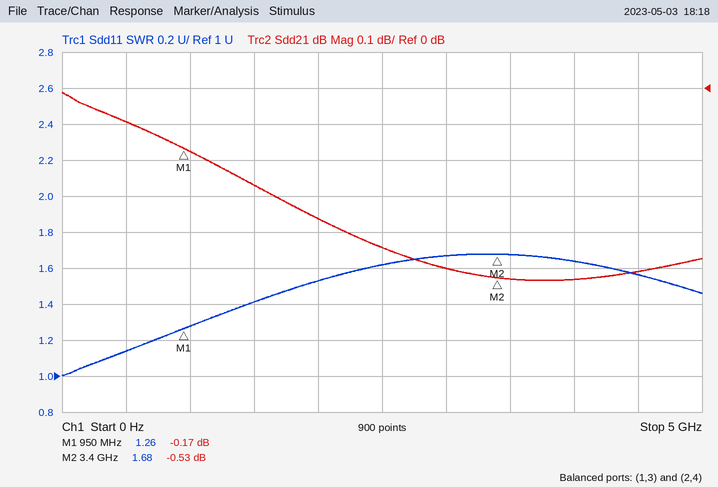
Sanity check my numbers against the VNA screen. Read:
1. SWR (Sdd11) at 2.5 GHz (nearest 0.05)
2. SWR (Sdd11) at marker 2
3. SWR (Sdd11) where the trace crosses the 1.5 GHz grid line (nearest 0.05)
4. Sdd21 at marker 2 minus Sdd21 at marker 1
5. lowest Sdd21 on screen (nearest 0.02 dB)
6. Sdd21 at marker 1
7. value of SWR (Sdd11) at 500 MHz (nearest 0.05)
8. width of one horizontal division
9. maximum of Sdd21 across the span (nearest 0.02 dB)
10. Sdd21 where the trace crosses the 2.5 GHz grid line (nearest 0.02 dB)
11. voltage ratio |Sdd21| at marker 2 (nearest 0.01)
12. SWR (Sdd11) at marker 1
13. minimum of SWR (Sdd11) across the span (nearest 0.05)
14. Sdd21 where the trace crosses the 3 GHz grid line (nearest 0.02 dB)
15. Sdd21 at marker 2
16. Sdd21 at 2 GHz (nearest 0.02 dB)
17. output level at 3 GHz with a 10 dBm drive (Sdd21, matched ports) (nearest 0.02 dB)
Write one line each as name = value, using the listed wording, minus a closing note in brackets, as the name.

SWR (Sdd11) at 2.5 GHz = 1.60
SWR (Sdd11) at marker 2 = 1.68
SWR (Sdd11) where the trace crosses the 1.5 GHz grid line = 1.40
Sdd21 at marker 2 minus Sdd21 at marker 1 = -0.36 dB
lowest Sdd21 on screen = -0.54 dB
Sdd21 at marker 1 = -0.17 dB
value of SWR (Sdd11) at 500 MHz = 1.15
width of one horizontal division = 500 MHz
maximum of Sdd21 across the span = -0.02 dB
Sdd21 where the trace crosses the 2.5 GHz grid line = -0.44 dB
voltage ratio |Sdd21| at marker 2 = 0.94
SWR (Sdd11) at marker 1 = 1.26
minimum of SWR (Sdd11) across the span = 1.00
Sdd21 where the trace crosses the 3 GHz grid line = -0.50 dB
Sdd21 at marker 2 = -0.53 dB
Sdd21 at 2 GHz = -0.36 dB
output level at 3 GHz with a 10 dBm drive (Sdd21, matched ports) = 9.50 dBm
